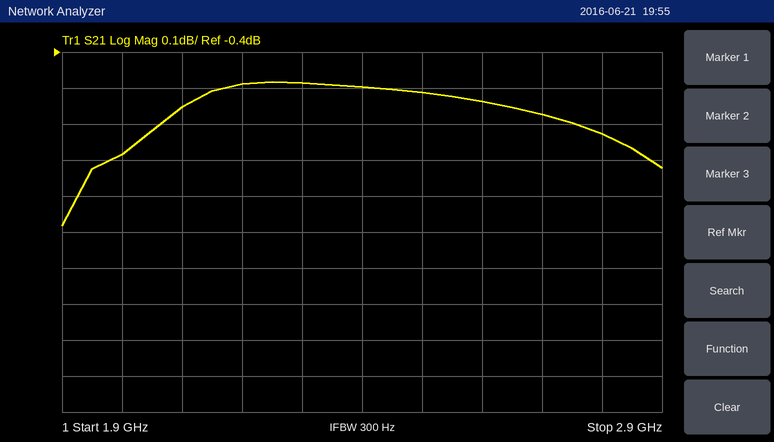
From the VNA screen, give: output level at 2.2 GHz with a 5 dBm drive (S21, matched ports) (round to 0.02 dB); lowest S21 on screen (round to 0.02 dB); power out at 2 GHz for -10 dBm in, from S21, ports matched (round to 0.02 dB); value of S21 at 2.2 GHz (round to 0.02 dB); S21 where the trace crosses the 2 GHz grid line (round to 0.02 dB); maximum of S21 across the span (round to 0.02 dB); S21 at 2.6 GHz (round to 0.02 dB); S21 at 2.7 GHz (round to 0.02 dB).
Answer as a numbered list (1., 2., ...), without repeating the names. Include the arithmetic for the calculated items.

1. 5 dBm + (-0.48 dB) = 4.52 dBm
2. -0.88 dB
3. -10 dBm + (-0.68 dB) = -10.68 dBm
4. -0.48 dB
5. -0.68 dB
6. -0.48 dB
7. -0.54 dB
8. -0.58 dB
